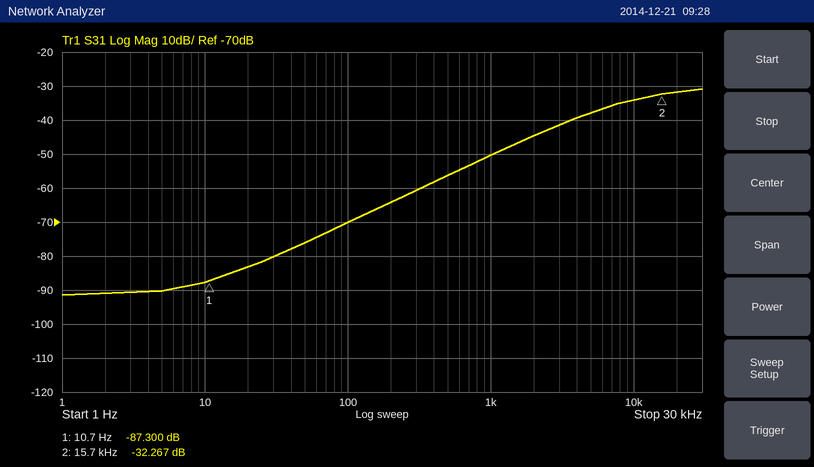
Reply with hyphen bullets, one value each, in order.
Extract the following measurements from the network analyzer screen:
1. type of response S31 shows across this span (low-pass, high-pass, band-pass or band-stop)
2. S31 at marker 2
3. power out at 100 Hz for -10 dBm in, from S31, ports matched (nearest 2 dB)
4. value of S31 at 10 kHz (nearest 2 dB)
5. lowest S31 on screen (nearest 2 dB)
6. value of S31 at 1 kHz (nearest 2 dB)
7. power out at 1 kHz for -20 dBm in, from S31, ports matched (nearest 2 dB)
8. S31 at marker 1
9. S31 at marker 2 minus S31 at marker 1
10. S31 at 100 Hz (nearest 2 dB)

- high-pass
- -32.267 dB
- -80 dBm
- -34 dB
- -92 dB
- -50 dB
- -70 dBm
- -87.300 dB
- 55.033 dB
- -70 dB
